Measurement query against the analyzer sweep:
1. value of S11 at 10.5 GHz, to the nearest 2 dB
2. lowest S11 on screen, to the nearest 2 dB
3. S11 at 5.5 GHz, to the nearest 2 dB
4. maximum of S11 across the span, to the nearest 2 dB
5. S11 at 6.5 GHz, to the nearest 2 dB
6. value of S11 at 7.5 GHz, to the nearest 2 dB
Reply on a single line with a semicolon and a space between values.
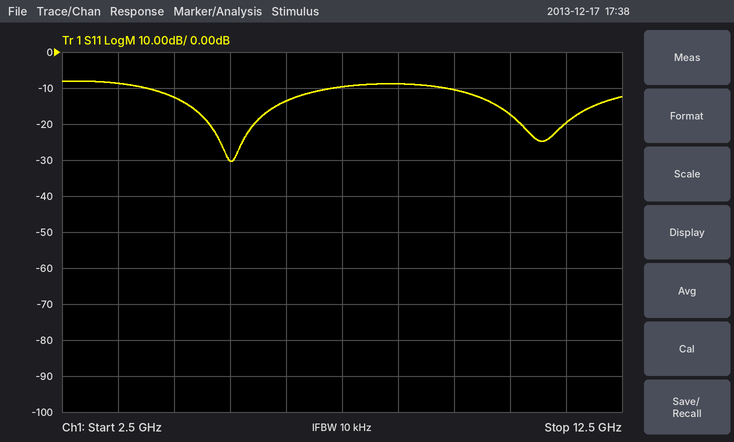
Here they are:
-18 dB; -30 dB; -30 dB; -8 dB; -14 dB; -10 dB
